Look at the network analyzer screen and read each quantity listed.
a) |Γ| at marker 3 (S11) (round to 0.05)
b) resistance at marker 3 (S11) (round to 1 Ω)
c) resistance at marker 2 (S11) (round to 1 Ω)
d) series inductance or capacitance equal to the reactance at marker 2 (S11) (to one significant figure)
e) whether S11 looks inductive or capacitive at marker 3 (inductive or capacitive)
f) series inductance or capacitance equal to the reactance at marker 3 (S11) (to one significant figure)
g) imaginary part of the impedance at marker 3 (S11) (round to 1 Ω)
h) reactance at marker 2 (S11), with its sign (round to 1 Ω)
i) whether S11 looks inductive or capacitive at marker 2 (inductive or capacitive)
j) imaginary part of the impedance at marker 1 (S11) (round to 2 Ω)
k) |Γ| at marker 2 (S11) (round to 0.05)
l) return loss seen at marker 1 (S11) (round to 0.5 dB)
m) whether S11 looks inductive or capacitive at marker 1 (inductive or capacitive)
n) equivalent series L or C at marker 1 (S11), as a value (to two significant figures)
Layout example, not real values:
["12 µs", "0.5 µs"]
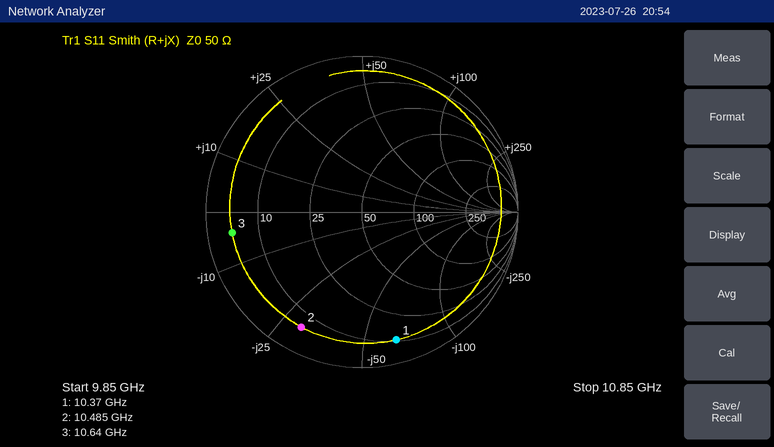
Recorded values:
["0.85", "4 Ω", "6 Ω", "500 fF", "capacitive", "4 pF", "-4 Ω", "-30 Ω", "capacitive", "-64 Ω", "0.85", "1.5 dB", "capacitive", "240 fF"]
